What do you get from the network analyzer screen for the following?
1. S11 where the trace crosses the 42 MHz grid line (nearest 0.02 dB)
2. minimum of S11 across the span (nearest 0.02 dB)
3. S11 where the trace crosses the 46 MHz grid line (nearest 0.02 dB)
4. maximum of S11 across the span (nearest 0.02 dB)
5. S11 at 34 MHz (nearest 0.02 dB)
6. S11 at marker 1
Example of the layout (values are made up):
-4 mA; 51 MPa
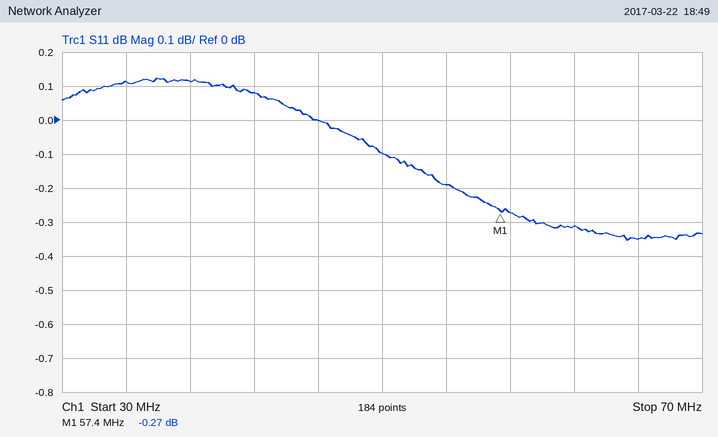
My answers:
0.08 dB; -0.36 dB; 0.00 dB; 0.12 dB; 0.12 dB; -0.27 dB
